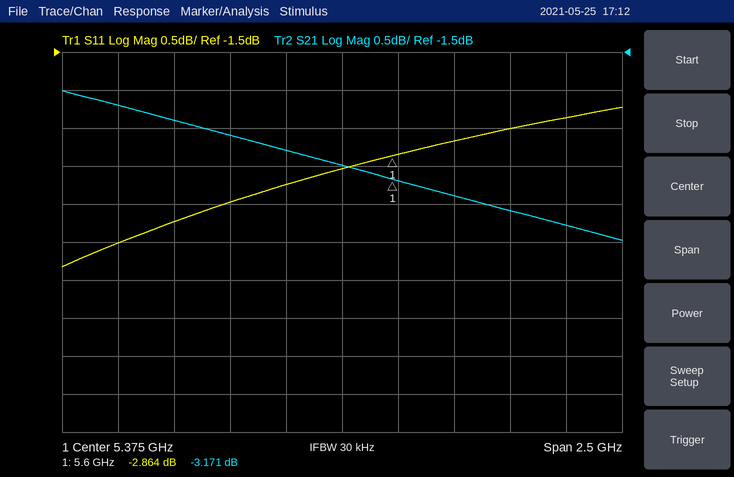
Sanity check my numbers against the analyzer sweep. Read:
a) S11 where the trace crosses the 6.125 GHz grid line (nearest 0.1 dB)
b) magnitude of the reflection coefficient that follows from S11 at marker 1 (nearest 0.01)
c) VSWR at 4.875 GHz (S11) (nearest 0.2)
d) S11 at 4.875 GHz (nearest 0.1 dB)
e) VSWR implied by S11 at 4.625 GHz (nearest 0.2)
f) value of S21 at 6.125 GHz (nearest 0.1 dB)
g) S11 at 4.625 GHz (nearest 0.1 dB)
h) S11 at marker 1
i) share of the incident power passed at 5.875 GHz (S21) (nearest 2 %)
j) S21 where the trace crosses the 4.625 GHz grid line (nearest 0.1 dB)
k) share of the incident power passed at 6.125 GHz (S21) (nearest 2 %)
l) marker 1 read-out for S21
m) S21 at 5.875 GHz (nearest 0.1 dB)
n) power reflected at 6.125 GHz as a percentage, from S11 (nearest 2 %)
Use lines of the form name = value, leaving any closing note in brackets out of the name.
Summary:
S11 where the trace crosses the 6.125 GHz grid line = -2.5 dB
magnitude of the reflection coefficient that follows from S11 at marker 1 = 0.72
VSWR at 4.875 GHz (S11) = 5.0
S11 at 4.875 GHz = -3.5 dB
VSWR implied by S11 at 4.625 GHz = 4.8
value of S21 at 6.125 GHz = -3.6 dB
S11 at 4.625 GHz = -3.7 dB
S11 at marker 1 = -2.864 dB
share of the incident power passed at 5.875 GHz (S21) = 46 %
S21 where the trace crosses the 4.625 GHz grid line = -2.4 dB
share of the incident power passed at 6.125 GHz (S21) = 44 %
marker 1 read-out for S21 = -3.171 dB
S21 at 5.875 GHz = -3.4 dB
power reflected at 6.125 GHz as a percentage, from S11 = 56 %
